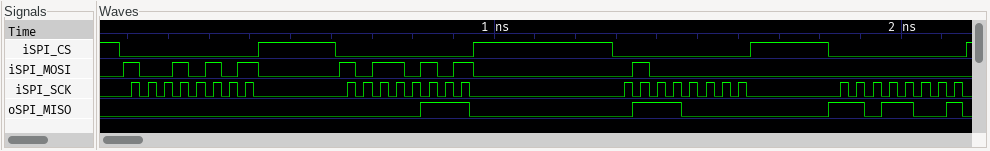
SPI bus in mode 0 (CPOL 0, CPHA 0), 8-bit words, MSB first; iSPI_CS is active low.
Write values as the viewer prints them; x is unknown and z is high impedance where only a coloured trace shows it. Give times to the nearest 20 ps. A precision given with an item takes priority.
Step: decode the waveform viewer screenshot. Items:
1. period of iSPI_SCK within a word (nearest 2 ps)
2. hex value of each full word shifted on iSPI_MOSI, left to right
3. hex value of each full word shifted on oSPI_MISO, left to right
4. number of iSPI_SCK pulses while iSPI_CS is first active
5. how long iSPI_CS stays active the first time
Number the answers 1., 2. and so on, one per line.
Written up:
1. 40 ps
2. 95, B5, 40, 00
3. 00, 07, 70, D9
4. 8
5. 340 ps
